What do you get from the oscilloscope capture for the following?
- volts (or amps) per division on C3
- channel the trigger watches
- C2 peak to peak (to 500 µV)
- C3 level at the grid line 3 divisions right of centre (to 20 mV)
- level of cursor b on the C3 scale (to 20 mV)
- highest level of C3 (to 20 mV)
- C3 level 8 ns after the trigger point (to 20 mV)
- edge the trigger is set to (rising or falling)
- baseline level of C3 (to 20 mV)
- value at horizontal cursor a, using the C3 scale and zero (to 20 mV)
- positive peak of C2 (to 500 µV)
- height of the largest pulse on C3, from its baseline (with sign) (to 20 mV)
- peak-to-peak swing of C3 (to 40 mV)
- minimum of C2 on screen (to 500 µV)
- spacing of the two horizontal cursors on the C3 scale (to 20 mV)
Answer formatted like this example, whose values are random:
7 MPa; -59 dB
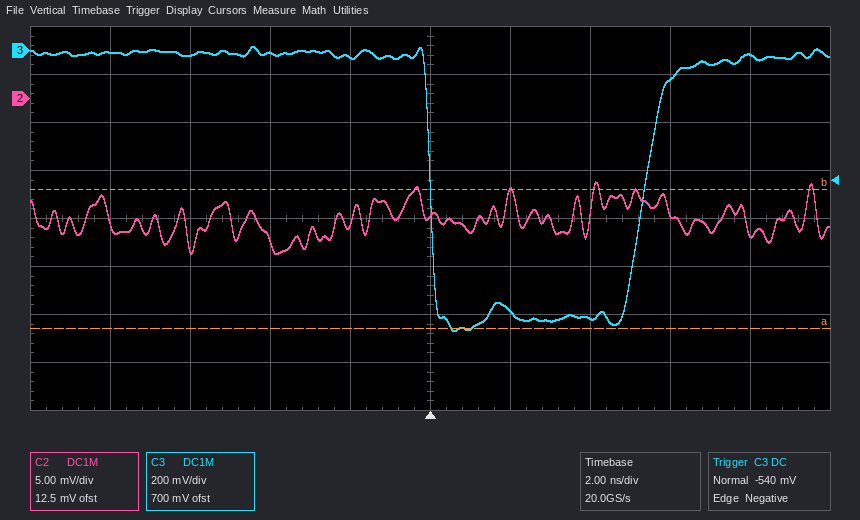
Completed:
200 mV; C3; 7.5 mV; -120 mV; -580 mV; 20 mV; -20 mV; falling; -20 mV; -1.16 V; -8.5 mV; -1.16 V; 1.20 V; -16.0 mV; 580 mV
